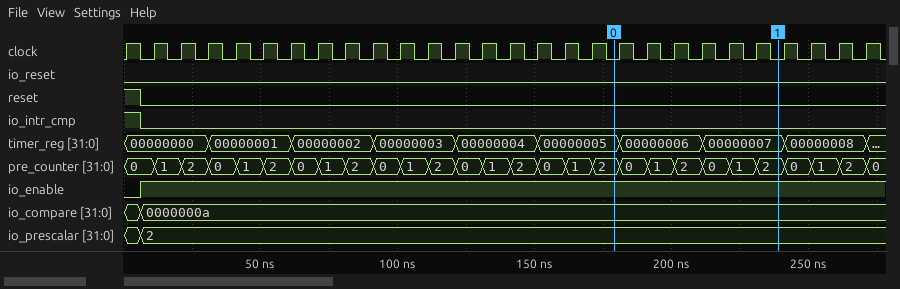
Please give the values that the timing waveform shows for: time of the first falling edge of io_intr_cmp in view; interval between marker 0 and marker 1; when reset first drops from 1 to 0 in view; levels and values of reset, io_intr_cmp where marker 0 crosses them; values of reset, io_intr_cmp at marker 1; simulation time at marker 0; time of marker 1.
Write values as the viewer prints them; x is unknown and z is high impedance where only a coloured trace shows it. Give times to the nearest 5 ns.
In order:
5 ns
60 ns
5 ns
reset=0, io_intr_cmp=0
reset=0, io_intr_cmp=0
180 ns
240 ns
